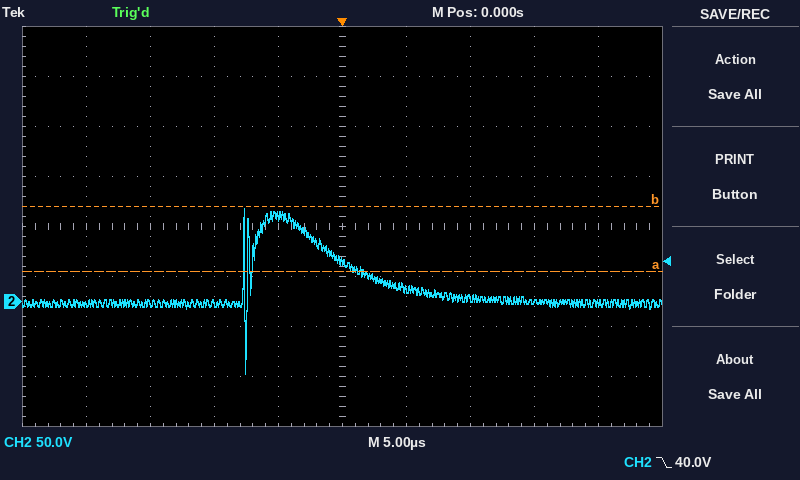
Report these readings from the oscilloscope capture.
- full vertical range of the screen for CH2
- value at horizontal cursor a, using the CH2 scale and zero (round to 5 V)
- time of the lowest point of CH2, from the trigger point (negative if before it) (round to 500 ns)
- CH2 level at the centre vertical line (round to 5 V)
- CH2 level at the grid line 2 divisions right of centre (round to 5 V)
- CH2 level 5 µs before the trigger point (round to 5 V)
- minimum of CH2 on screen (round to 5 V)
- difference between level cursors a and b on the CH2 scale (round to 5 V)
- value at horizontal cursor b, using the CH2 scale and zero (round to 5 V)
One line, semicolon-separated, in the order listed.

400 V; 30 V; -7.5 µs; 40 V; 5 V; 85 V; -70 V; 65 V; 95 V
